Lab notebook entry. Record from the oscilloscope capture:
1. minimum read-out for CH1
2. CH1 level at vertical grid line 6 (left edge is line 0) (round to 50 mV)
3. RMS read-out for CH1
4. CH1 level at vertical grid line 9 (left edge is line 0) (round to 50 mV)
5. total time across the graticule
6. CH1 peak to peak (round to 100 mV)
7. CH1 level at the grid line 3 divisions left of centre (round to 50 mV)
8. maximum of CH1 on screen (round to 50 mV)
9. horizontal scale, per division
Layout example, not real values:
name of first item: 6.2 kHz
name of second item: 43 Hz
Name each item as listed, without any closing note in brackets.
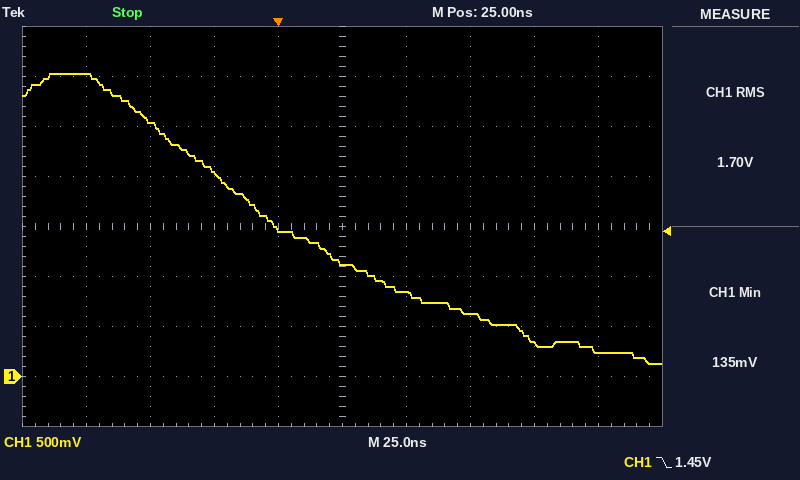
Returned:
minimum read-out for CH1: 135 mV
CH1 level at vertical grid line 6 (left edge is line 0): 850 mV
RMS read-out for CH1: 1.70 V
CH1 level at vertical grid line 9 (left edge is line 0): 250 mV
total time across the graticule: 250 ns
CH1 peak to peak: 2.90 V
CH1 level at the grid line 3 divisions left of centre: 2.55 V
maximum of CH1 on screen: 3.05 V
horizontal scale, per division: 25 ns
